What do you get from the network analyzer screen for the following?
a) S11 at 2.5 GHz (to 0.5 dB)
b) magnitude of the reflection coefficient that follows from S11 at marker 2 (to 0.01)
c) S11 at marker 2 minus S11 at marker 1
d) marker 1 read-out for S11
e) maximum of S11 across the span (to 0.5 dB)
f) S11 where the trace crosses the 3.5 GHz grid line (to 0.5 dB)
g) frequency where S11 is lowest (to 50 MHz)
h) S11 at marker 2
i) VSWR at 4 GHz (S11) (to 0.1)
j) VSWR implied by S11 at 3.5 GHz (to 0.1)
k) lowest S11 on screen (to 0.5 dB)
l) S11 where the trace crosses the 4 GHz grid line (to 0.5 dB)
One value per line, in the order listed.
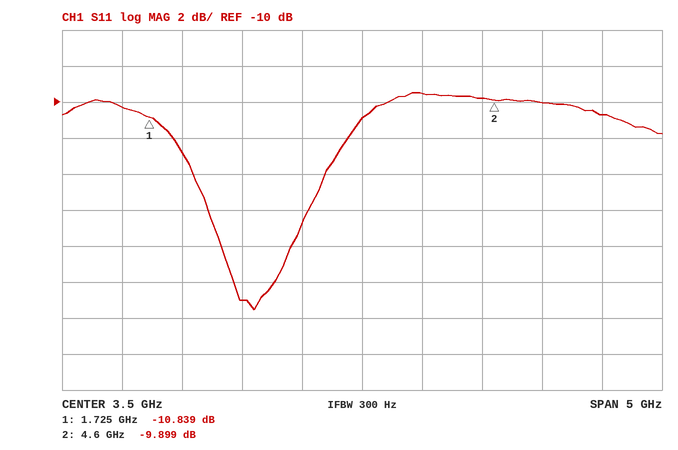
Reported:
-21.0 dB
0.32
0.940 dB
-10.839 dB
-9.5 dB
-11.0 dB
2.60 GHz
-9.899 dB
2.0
1.8
-21.5 dB
-9.5 dB
